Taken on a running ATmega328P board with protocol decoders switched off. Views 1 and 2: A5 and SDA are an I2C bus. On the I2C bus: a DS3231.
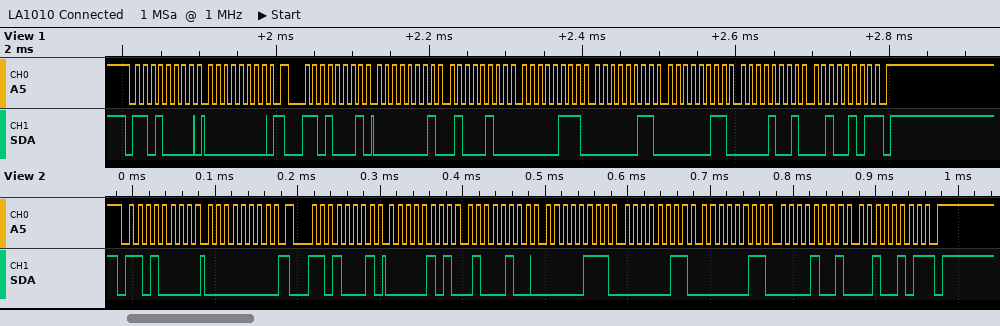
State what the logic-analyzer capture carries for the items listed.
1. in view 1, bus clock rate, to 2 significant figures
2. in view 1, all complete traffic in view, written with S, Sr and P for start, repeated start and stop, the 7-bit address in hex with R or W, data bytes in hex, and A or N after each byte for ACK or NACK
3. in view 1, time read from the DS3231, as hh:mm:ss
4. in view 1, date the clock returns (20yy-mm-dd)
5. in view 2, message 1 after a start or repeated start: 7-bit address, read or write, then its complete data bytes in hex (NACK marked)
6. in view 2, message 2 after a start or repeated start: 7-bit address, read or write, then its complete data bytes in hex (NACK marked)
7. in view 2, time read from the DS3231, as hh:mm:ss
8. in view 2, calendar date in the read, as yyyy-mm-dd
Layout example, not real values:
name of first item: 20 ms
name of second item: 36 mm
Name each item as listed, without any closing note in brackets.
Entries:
in view 1, bus clock rate, to 2 significant figures: 100 kHz
in view 1, all complete traffic in view, written with S, Sr and P for start, repeated start and stop, the 7-bit address in hex with R or W, data bytes in hex, and A or N after each byte for ACK or NACK: S 68W A 00 A Sr 68R A 01 A 44 A 07 A 03 A 03 A 09 A 25 N P
in view 1, time read from the DS3231, as hh:mm:ss: 07:44:01
in view 1, date the clock returns: 2025-09-03
in view 2, message 1 after a start or repeated start: 7-bit address, read or write, then its complete data bytes in hex: 0x68 write: 00
in view 2, message 2 after a start or repeated start: 7-bit address, read or write, then its complete data bytes in hex: 0x68 read: 05 44 07 03 03 09 25 NACK
in view 2, time read from the DS3231, as hh:mm:ss: 07:44:05
in view 2, calendar date in the read, as yyyy-mm-dd: 2025-09-03
